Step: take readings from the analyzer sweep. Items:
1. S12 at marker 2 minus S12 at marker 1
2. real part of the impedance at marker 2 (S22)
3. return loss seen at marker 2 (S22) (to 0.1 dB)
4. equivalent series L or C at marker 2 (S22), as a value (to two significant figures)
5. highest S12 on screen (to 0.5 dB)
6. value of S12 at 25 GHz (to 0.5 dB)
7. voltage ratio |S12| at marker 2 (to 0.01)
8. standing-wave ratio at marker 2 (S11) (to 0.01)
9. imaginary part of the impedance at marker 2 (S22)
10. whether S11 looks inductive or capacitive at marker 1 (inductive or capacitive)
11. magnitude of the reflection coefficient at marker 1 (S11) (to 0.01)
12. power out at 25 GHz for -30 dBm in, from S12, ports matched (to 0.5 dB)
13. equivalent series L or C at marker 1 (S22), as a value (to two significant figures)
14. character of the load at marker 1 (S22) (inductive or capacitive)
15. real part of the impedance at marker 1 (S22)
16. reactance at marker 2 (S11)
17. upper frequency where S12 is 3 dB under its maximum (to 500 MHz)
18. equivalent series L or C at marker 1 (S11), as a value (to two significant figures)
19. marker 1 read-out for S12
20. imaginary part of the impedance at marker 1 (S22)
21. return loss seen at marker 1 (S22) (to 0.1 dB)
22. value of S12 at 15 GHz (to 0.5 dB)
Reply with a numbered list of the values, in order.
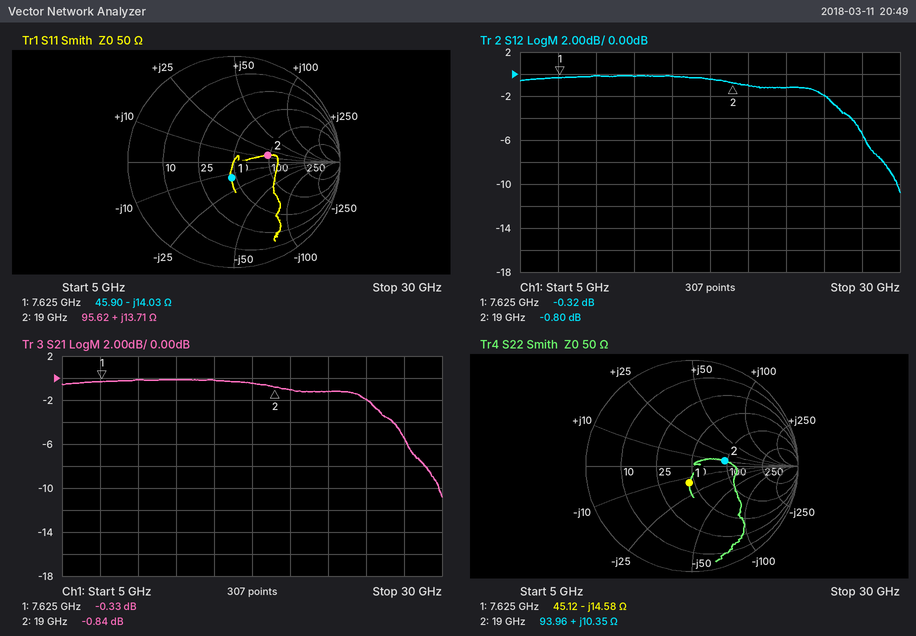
1. -0.48 dB
2. 93.96 Ω
3. 10.1 dB
4. 87 pH
5. 0.0 dB
6. -2.0 dB
7. 0.91
8. 1.97
9. +10.35 Ω
10. capacitive
11. 0.15
12. -32.0 dBm
13. 1.4 pF
14. capacitive
15. 45.12 Ω
16. +13.71 Ω
17. 26.0 GHz
18. 1.5 pF
19. -0.32 dB
20. -14.58 Ω
21. 15.9 dB
22. 0.0 dB
